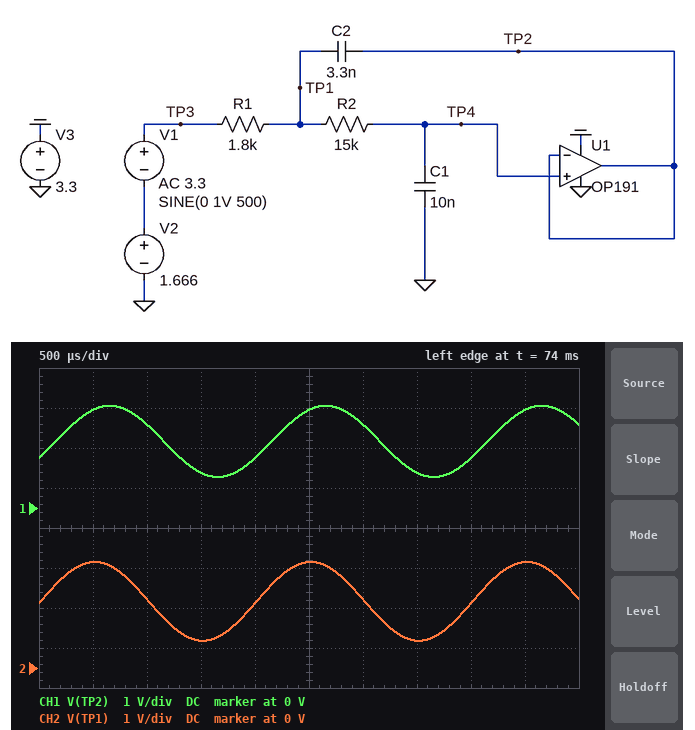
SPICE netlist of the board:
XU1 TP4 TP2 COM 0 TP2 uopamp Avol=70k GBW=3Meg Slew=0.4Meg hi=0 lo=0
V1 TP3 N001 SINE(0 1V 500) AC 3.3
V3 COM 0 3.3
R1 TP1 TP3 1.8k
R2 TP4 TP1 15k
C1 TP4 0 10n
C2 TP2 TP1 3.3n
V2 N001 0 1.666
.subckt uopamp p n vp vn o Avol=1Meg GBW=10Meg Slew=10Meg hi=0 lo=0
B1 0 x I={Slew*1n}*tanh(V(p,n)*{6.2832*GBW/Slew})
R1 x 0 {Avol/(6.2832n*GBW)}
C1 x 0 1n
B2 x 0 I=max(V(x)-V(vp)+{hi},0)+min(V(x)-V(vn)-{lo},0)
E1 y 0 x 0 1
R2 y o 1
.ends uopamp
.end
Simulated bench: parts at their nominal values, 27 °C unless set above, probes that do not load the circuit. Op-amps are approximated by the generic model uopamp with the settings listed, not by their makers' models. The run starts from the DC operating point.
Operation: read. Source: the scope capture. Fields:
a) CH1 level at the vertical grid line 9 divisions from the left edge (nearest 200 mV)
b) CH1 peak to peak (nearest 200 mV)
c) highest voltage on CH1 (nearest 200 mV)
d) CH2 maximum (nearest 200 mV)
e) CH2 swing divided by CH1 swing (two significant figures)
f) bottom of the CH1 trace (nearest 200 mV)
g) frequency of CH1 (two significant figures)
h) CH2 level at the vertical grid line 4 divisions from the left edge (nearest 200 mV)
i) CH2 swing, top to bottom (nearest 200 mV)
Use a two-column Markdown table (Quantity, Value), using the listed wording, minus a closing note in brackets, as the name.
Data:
| Quantity | Value |
|---|---|
| CH1 level at the vertical grid line 9 divisions from the left edge | 2.4 V |
| CH1 peak to peak | 1.8 V |
| highest voltage on CH1 | 2.6 V |
| CH2 maximum | 2.6 V |
| CH2 swing divided by CH1 swing | 1.1 |
| bottom of the CH1 trace | 800 mV |
| frequency of CH1 | 500 Hz |
| CH2 level at the vertical grid line 4 divisions from the left edge | 1.6 V |
| CH2 swing, top to bottom | 2.0 V |
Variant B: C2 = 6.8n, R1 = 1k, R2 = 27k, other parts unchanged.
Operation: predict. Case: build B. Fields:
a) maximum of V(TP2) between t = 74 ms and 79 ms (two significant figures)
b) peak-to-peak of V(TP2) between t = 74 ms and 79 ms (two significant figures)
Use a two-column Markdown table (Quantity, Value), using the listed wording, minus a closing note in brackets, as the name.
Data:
| Quantity | Value |
|---|---|
| maximum of V(TP2) between t = 74 ms and 79 ms | 2.4 V |
| peak-to-peak of V(TP2) between t = 74 ms and 79 ms | 1.5 V |
